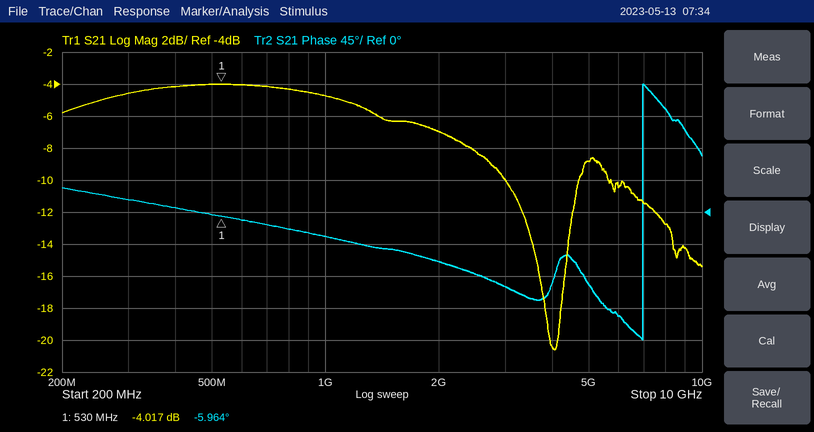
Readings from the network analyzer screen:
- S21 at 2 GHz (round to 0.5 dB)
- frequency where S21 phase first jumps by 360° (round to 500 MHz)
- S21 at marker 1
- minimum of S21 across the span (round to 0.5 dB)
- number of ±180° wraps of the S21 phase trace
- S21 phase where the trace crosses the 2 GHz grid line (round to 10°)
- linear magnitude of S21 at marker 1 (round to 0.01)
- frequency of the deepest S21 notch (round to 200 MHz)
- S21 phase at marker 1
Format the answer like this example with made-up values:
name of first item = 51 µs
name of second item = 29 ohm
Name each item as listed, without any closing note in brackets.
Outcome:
S21 at 2 GHz = -7.0 dB
frequency where S21 phase first jumps by 360° = 7.0 GHz
S21 at marker 1 = -4.017 dB
minimum of S21 across the span = -20.5 dB
number of ±180° wraps of the S21 phase trace = 1
S21 phase where the trace crosses the 2 GHz grid line = -70°
linear magnitude of S21 at marker 1 = 0.63
frequency of the deepest S21 notch = 4.0 GHz
S21 phase at marker 1 = -5.964°
